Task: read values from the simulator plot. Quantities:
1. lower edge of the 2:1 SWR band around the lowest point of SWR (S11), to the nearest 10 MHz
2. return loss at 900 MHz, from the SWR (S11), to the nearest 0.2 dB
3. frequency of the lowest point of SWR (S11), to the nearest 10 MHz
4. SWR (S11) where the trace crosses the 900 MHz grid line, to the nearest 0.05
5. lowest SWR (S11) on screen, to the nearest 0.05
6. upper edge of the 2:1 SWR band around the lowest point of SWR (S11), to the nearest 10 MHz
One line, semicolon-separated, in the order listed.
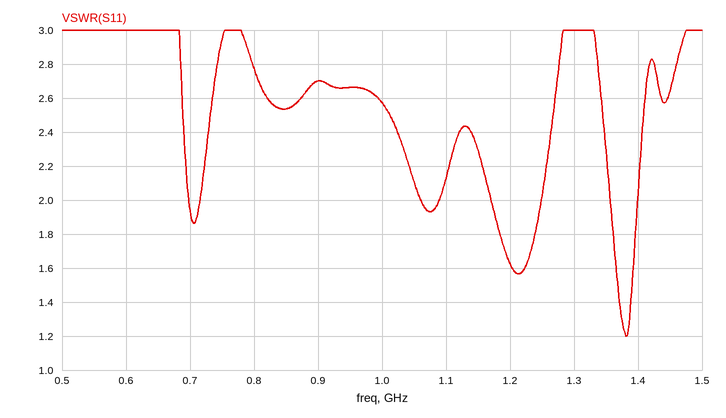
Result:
1.36 GHz; 6.8 dB; 1.38 GHz; 2.70; 1.20; 1.40 GHz
